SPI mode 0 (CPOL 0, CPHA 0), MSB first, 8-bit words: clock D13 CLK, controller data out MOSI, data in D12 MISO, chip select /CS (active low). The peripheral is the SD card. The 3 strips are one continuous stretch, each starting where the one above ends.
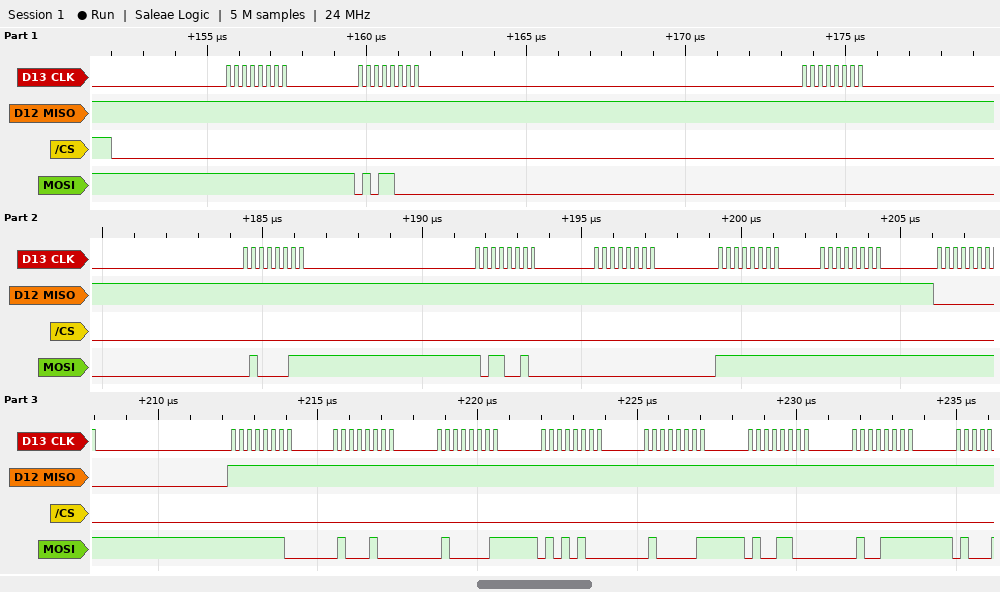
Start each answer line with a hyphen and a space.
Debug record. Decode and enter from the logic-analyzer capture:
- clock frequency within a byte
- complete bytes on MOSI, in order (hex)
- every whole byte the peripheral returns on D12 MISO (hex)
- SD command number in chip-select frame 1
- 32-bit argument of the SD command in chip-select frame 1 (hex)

- 4 MHz
- 0xFF 0x58 0x00 0x43 0xB2 0x00 0xFF 0xFF 0xFF 0xFE 0x44 0x41 0x54 0x41 0x4C 0x4F
- 0xFF 0xFF 0xFF 0xFF 0xFF 0xFF 0xFF 0xFF 0x00 0xFF 0xFF 0xFF 0xFF 0xFF 0xFF 0xFF
- CMD24
- 0x0043B200
